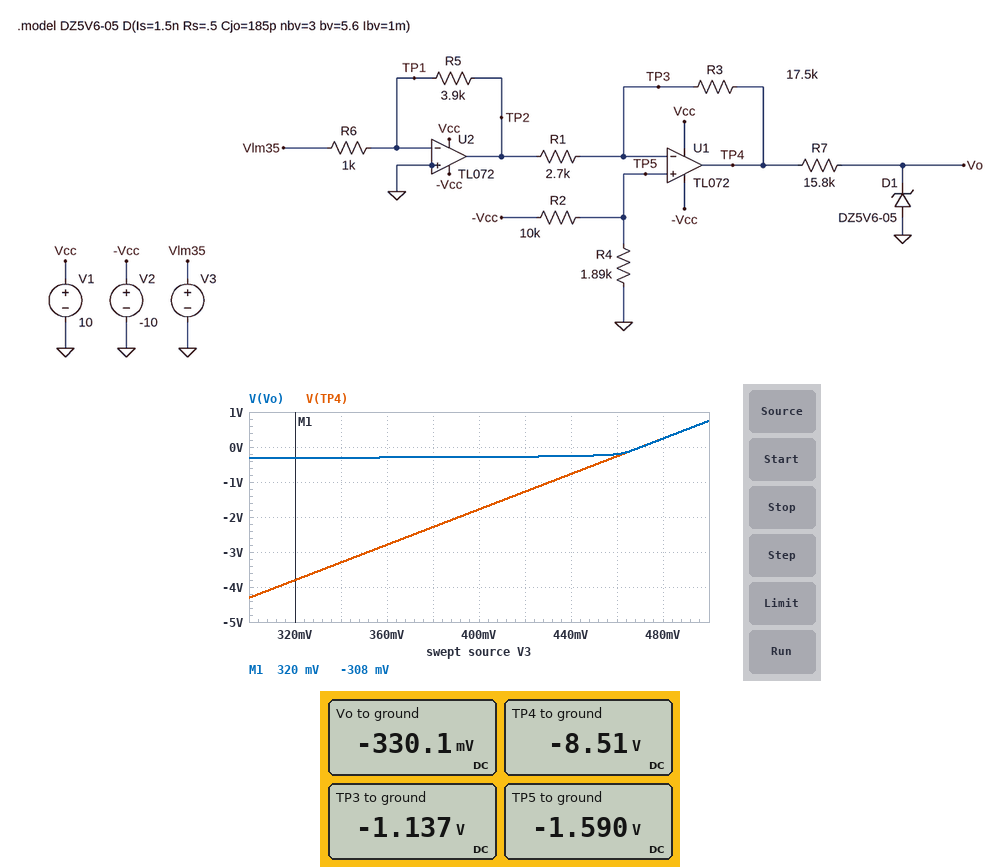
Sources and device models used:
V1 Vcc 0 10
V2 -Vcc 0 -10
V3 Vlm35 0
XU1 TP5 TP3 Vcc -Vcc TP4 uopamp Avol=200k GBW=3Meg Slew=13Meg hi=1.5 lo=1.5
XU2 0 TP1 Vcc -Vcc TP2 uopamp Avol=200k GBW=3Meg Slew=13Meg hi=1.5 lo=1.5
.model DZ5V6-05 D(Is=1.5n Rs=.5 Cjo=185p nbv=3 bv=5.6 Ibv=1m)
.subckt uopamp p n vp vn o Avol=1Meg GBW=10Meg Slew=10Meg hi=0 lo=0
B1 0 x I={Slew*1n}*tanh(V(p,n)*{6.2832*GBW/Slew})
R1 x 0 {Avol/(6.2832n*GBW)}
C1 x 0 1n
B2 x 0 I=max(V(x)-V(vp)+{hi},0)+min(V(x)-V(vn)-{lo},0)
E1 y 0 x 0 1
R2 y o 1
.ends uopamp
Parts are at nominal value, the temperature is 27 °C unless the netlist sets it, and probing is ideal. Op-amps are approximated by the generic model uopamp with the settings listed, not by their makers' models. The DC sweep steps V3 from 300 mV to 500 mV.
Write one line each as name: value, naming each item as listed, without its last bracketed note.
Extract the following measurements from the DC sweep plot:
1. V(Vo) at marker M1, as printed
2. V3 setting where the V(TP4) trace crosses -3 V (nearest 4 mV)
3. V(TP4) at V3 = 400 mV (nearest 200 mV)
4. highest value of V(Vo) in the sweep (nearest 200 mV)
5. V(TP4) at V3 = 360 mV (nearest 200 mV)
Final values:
V(Vo) at marker M1, as printed: -308 mV
V3 setting where the V(TP4) trace crosses -3 V: 352 mV
V(TP4) at V3 = 400 mV: -1.8 V
highest value of V(Vo) in the sweep: 800 mV
V(TP4) at V3 = 360 mV: -2.8 V
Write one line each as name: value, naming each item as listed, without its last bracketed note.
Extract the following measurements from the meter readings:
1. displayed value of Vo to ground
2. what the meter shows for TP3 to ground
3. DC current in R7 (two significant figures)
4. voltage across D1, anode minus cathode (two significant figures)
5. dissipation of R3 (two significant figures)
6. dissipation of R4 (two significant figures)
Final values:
displayed value of Vo to ground: -330.1 mV
what the meter shows for TP3 to ground: -1.137 V
DC current in R7: 520 µA
voltage across D1, anode minus cathode: 330 mV
dissipation of R3: 3.1 mW
dissipation of R4: 1.3 mW
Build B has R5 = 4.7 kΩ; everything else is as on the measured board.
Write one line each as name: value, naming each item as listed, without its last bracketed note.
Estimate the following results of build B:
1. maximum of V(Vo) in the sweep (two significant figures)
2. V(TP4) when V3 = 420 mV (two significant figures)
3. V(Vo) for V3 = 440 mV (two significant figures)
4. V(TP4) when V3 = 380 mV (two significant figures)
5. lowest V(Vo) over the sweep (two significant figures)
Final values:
maximum of V(Vo) in the sweep: 3.3 V
V(TP4) when V3 = 420 mV: 900 mV
V(Vo) for V3 = 440 mV: 1.5 V
V(TP4) when V3 = 380 mV: -320 mV
lowest V(Vo) over the sweep: -300 mV
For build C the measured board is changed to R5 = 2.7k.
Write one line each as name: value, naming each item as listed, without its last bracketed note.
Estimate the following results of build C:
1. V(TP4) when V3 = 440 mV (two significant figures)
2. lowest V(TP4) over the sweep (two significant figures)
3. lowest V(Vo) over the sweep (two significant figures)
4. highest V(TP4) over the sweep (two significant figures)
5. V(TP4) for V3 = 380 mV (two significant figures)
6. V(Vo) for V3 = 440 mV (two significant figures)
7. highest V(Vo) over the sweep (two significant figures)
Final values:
V(TP4) when V3 = 440 mV: -4.2 V
lowest V(TP4) over the sweep: -6.6 V
lowest V(Vo) over the sweep: -320 mV
highest V(TP4) over the sweep: -3.1 V
V(TP4) for V3 = 380 mV: -5.2 V
V(Vo) for V3 = 440 mV: -310 mV
highest V(Vo) over the sweep: -300 mV
